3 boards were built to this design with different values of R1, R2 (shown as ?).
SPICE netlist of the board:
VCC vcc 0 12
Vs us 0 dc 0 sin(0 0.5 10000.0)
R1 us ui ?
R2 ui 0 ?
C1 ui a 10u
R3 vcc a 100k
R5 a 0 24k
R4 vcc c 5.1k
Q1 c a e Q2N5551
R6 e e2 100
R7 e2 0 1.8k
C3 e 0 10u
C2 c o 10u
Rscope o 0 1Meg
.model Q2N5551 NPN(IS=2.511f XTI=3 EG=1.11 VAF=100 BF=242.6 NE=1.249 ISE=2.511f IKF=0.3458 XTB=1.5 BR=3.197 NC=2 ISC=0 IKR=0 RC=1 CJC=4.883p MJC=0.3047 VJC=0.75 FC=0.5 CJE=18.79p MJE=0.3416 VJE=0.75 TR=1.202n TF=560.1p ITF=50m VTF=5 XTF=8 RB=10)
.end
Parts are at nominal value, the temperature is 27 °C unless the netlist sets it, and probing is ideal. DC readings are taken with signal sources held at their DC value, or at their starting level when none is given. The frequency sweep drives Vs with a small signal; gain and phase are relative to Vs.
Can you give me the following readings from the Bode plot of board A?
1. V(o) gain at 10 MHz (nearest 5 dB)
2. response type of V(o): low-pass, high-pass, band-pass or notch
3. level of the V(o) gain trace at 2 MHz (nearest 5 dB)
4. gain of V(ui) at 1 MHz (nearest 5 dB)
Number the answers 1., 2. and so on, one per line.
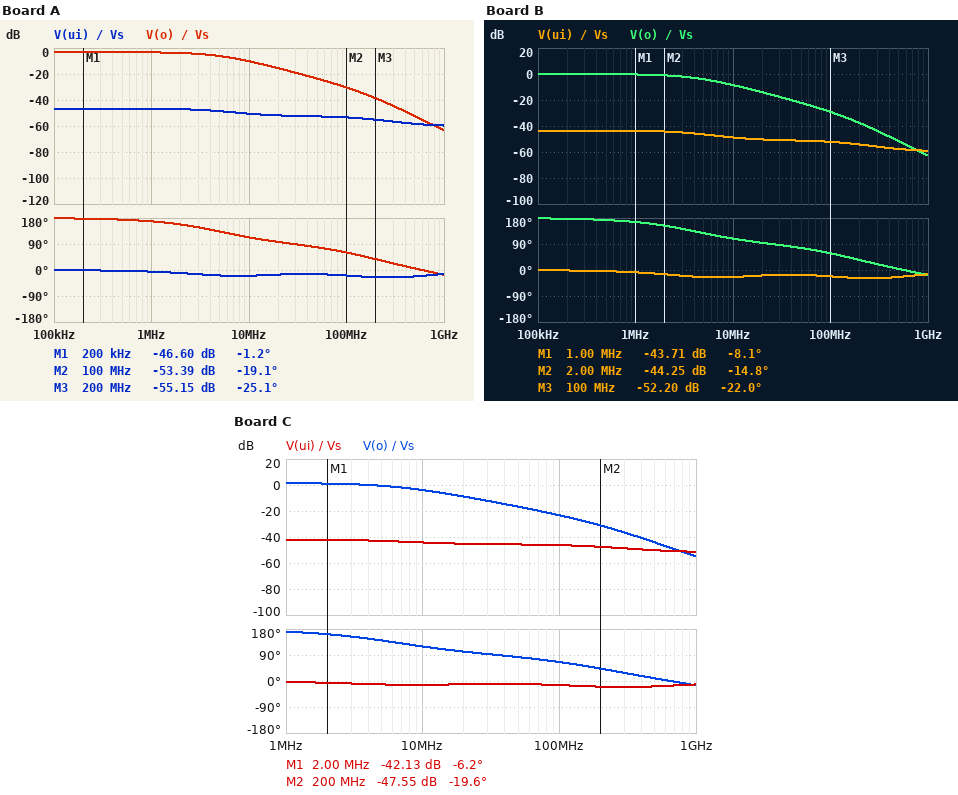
1. -10 dB
2. low-pass
3. -5 dB
4. -45 dB
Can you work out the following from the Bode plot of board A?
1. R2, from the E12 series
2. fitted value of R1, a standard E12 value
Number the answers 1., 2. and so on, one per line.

1. 39 Ω
2. 8.2 kΩ
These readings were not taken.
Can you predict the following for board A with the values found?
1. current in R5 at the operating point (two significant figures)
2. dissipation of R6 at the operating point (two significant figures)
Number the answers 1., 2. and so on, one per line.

1. 91 µA
2. 63 µW
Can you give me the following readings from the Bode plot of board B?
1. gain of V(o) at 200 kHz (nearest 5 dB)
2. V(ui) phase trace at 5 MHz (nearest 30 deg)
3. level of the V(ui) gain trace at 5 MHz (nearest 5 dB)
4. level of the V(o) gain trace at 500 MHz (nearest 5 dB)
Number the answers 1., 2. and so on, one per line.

1. 0 dB
2. -30 deg
3. -45 dB
4. -50 dB
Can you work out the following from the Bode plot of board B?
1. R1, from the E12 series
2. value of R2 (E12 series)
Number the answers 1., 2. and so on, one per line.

1. 8.2 kΩ
2. 56 Ω
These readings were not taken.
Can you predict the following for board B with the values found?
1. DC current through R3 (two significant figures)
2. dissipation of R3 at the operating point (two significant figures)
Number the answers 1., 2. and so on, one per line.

1. 98 µA
2. 960 µW
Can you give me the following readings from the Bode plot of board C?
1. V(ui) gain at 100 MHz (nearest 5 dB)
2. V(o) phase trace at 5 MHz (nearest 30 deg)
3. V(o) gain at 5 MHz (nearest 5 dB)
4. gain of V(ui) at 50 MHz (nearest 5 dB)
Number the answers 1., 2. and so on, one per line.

1. -45 dB
2. 150 deg
3. 0 dB
4. -45 dB
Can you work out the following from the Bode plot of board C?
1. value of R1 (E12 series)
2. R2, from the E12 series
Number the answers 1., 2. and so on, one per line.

1. 2.7 kΩ
2. 22 Ω
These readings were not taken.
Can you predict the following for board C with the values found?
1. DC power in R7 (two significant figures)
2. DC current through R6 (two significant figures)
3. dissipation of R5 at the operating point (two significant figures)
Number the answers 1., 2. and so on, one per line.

1. 1.1 mW
2. 790 µA
3. 200 µW
